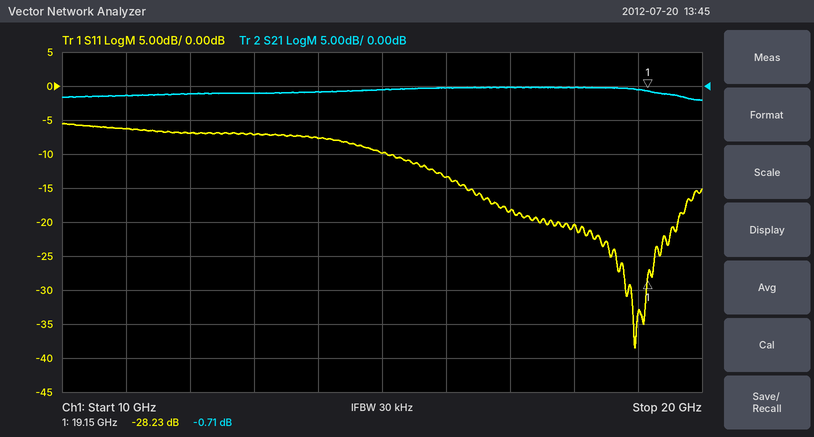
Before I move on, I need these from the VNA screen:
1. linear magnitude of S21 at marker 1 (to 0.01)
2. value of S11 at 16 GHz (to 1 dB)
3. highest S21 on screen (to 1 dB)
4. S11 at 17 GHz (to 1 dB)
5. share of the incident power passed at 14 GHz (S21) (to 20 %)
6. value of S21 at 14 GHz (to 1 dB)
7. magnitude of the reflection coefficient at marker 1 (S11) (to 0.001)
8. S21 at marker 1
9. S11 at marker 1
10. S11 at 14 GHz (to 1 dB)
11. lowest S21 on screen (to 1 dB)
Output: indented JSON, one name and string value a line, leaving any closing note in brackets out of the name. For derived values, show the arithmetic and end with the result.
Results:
{
  "linear magnitude of S21 at marker 1": "10^(-0.71/20) ≈ 0.92",
  "value of S11 at 16 GHz": "-13 dB",
  "highest S21 on screen": "0 dB",
  "S11 at 17 GHz": "-18 dB",
  "share of the incident power passed at 14 GHz (S21)": "10^(-1/10) ≈ 79.4 %, so 80 % to the nearest 20 %",
  "value of S21 at 14 GHz": "-1 dB",
  "magnitude of the reflection coefficient at marker 1 (S11)": "10^(-28.23/20) ≈ 0.039",
  "S21 at marker 1": "-0.71 dB",
  "S11 at marker 1": "-28.23 dB",
  "S11 at 14 GHz": "-8 dB",
  "lowest S21 on screen": "-2 dB"
}
